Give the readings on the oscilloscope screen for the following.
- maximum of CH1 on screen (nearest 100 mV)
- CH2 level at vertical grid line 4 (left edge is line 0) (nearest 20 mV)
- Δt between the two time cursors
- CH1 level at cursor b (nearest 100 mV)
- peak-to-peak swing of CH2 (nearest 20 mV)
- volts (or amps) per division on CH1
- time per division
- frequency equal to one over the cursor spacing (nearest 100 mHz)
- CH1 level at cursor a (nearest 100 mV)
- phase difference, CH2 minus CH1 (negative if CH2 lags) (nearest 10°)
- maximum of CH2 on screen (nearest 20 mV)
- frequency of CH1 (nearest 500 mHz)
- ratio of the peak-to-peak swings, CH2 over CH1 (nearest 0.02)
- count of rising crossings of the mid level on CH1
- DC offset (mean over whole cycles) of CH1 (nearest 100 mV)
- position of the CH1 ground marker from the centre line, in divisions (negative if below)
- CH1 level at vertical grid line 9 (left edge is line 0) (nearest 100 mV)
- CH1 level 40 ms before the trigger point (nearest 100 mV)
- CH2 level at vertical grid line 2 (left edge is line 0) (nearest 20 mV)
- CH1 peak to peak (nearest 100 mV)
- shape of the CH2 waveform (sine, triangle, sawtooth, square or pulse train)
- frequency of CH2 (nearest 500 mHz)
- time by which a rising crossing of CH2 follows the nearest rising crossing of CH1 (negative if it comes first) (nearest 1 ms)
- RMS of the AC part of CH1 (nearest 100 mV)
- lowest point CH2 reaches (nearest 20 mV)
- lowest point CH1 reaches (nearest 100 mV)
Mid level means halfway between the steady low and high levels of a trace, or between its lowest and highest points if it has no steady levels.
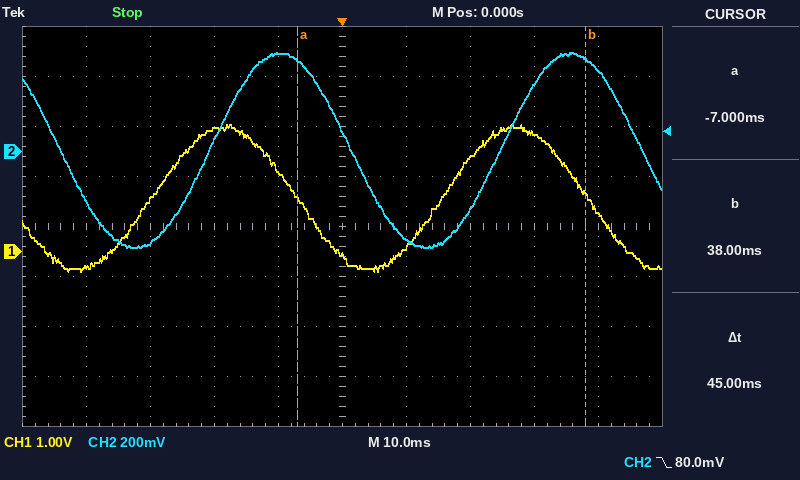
2.5 V
400 mV
45 ms
1.1 V
780 mV
1 V
10 ms
22.2 Hz
1.1 V
-70°
400 mV
22.0 Hz
0.26
2
1.1 V
-0.5 div
800 mV
-300 mV
-360 mV
2.9 V
sine
22.0 Hz
+9 ms
1.0 V
-380 mV
-400 mV
